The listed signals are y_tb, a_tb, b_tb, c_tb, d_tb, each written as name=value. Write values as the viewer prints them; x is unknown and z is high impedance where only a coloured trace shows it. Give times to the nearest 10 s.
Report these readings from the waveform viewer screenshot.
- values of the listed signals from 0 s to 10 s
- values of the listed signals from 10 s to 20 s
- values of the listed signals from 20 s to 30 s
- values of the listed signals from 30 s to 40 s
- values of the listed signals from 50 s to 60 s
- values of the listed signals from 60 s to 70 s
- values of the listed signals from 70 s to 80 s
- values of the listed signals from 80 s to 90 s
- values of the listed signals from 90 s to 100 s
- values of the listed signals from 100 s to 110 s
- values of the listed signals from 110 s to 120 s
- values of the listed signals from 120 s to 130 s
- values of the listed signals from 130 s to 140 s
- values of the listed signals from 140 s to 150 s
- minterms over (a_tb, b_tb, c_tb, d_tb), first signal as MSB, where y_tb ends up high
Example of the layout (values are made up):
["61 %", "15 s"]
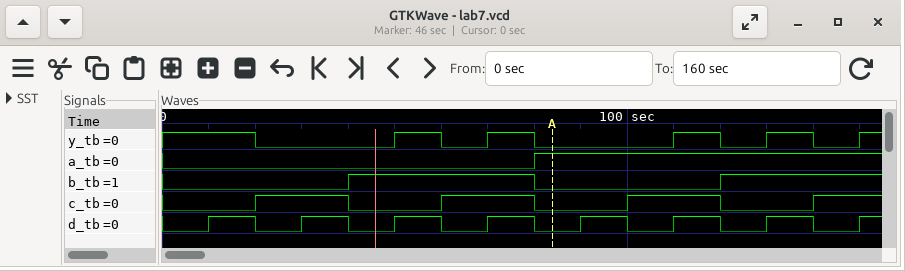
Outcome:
["y_tb=1, a_tb=0, b_tb=0, c_tb=0, d_tb=0", "y_tb=1, a_tb=0, b_tb=0, c_tb=0, d_tb=1", "y_tb=0, a_tb=0, b_tb=0, c_tb=1, d_tb=0", "y_tb=0, a_tb=0, b_tb=0, c_tb=1, d_tb=1", "y_tb=1, a_tb=0, b_tb=1, c_tb=0, d_tb=1", "y_tb=0, a_tb=0, b_tb=1, c_tb=1, d_tb=0", "y_tb=1, a_tb=0, b_tb=1, c_tb=1, d_tb=1", "y_tb=0, a_tb=1, b_tb=0, c_tb=0, d_tb=0", "y_tb=0, a_tb=1, b_tb=0, c_tb=0, d_tb=1", "y_tb=0, a_tb=1, b_tb=0, c_tb=1, d_tb=0", "y_tb=1, a_tb=1, b_tb=0, c_tb=1, d_tb=1", "y_tb=0, a_tb=1, b_tb=1, c_tb=0, d_tb=0", "y_tb=1, a_tb=1, b_tb=1, c_tb=0, d_tb=1", "y_tb=0, a_tb=1, b_tb=1, c_tb=1, d_tb=0", "0, 1, 5, 7, 11, 13, 15"]
